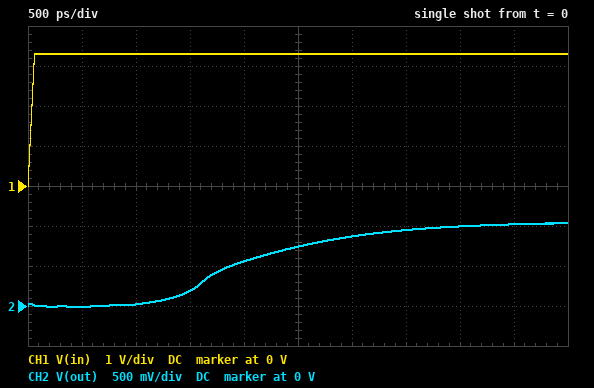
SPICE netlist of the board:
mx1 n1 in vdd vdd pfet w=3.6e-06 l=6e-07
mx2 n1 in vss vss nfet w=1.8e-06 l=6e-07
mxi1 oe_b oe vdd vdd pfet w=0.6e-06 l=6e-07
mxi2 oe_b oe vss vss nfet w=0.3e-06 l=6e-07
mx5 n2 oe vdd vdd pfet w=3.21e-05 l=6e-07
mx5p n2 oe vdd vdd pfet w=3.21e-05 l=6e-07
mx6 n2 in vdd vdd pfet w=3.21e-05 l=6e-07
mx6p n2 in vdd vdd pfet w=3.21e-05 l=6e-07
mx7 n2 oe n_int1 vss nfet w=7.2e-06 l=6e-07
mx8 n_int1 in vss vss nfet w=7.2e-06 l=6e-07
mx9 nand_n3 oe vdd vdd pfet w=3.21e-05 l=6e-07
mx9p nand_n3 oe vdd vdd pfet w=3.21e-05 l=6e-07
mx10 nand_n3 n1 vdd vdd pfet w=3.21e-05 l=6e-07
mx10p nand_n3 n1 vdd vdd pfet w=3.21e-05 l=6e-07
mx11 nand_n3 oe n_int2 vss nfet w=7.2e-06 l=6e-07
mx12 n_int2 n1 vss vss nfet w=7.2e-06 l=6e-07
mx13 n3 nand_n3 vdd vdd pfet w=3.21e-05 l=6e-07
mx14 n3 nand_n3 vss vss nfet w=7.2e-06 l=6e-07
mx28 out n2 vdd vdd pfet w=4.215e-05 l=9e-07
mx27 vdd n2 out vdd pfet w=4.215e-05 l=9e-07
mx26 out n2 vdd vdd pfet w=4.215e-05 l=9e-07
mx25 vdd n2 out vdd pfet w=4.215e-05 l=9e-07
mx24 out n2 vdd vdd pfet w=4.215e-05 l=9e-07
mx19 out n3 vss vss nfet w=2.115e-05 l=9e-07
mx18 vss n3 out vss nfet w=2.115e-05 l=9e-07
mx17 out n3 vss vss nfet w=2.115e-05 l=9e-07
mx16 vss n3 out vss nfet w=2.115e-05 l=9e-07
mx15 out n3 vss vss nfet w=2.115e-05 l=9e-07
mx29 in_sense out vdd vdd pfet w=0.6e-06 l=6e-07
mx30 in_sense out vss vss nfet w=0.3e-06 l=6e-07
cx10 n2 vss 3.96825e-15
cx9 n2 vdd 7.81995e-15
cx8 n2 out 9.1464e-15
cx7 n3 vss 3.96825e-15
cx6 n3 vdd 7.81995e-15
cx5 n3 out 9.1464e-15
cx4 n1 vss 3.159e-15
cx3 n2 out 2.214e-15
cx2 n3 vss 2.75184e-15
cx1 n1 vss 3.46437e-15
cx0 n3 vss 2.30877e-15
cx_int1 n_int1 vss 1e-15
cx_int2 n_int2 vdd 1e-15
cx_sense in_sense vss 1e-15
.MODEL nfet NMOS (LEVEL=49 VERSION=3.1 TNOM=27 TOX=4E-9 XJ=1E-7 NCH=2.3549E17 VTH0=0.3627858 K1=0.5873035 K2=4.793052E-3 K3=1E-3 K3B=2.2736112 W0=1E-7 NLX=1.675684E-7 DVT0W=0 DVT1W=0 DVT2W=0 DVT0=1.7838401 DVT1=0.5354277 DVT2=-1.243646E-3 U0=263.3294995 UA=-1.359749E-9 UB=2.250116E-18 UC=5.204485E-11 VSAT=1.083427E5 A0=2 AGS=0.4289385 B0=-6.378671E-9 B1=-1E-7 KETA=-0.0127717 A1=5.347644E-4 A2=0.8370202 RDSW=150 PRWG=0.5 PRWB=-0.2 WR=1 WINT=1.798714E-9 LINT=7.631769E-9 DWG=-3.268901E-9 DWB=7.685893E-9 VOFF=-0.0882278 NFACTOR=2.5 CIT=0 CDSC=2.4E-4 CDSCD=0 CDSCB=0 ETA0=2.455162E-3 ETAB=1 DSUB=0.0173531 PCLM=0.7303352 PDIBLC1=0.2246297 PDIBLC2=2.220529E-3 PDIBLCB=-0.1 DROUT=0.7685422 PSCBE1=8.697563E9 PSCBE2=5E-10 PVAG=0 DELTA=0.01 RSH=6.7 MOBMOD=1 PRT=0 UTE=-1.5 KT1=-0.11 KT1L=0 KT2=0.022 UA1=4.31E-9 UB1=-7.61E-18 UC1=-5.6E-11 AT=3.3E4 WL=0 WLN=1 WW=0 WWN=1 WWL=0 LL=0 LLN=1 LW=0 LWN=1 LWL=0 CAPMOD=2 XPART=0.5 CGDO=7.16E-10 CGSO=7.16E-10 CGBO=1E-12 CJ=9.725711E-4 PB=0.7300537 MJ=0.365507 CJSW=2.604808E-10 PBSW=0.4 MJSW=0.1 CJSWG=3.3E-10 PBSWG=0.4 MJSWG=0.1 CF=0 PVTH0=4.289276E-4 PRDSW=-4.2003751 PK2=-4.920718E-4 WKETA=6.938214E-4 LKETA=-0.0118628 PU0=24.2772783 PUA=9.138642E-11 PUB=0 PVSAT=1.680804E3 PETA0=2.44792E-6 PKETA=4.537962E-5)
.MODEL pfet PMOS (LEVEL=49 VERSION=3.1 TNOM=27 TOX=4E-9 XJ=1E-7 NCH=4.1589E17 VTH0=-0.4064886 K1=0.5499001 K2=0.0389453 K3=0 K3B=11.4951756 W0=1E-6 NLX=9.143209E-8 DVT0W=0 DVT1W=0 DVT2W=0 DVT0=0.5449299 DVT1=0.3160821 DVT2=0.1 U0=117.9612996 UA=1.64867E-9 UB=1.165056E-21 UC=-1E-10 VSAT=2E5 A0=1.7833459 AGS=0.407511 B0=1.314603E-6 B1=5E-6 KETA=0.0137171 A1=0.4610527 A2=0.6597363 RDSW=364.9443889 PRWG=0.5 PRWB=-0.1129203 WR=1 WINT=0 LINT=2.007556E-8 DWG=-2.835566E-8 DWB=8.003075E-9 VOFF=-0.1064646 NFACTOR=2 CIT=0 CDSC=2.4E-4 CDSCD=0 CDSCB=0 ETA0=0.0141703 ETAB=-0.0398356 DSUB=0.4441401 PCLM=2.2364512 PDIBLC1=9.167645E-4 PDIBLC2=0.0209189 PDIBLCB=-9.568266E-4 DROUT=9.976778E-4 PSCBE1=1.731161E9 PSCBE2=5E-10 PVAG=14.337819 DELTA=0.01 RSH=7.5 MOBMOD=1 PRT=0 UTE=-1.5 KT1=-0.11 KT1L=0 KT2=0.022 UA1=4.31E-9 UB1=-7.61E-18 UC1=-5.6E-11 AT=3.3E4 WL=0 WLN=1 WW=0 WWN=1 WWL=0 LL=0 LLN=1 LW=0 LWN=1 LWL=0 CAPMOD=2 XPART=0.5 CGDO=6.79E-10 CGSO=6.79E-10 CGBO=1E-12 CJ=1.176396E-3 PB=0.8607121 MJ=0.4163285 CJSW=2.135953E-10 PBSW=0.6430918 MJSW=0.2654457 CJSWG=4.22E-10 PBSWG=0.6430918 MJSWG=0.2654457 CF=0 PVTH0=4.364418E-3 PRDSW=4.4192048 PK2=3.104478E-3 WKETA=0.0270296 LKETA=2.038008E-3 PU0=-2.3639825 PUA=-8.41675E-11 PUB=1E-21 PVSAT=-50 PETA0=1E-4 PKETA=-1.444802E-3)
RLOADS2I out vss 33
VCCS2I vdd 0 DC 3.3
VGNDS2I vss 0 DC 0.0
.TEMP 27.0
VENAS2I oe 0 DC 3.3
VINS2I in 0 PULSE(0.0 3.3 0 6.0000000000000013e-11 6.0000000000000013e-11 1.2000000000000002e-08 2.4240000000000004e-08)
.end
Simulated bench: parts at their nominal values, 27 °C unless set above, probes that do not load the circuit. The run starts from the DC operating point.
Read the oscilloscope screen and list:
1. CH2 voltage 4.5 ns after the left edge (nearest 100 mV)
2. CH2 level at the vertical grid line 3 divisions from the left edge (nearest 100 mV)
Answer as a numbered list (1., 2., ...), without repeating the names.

1. 1.0 V
2. 200 mV
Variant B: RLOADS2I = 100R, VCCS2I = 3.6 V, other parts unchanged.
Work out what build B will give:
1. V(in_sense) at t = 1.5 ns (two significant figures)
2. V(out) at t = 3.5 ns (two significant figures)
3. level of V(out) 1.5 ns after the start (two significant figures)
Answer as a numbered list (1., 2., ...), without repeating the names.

1. 3.6 V
2. 2.3 V
3. 320 mV
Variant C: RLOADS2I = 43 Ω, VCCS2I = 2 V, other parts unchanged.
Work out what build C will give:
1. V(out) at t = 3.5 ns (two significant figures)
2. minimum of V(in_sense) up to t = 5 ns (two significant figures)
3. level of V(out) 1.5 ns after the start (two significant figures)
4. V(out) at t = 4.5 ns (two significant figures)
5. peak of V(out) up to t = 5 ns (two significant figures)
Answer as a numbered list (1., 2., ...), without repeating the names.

1. 460 mV
2. 2.0 V
3. 120 mV
4. 490 mV
5. 500 mV
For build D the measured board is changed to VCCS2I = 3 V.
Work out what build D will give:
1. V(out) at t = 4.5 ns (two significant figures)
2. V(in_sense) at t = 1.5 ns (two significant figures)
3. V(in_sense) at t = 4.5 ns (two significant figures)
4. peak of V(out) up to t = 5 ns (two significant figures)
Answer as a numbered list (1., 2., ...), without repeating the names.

1. 860 mV
2. 3.0 V
3. 2.9 V
4. 870 mV
